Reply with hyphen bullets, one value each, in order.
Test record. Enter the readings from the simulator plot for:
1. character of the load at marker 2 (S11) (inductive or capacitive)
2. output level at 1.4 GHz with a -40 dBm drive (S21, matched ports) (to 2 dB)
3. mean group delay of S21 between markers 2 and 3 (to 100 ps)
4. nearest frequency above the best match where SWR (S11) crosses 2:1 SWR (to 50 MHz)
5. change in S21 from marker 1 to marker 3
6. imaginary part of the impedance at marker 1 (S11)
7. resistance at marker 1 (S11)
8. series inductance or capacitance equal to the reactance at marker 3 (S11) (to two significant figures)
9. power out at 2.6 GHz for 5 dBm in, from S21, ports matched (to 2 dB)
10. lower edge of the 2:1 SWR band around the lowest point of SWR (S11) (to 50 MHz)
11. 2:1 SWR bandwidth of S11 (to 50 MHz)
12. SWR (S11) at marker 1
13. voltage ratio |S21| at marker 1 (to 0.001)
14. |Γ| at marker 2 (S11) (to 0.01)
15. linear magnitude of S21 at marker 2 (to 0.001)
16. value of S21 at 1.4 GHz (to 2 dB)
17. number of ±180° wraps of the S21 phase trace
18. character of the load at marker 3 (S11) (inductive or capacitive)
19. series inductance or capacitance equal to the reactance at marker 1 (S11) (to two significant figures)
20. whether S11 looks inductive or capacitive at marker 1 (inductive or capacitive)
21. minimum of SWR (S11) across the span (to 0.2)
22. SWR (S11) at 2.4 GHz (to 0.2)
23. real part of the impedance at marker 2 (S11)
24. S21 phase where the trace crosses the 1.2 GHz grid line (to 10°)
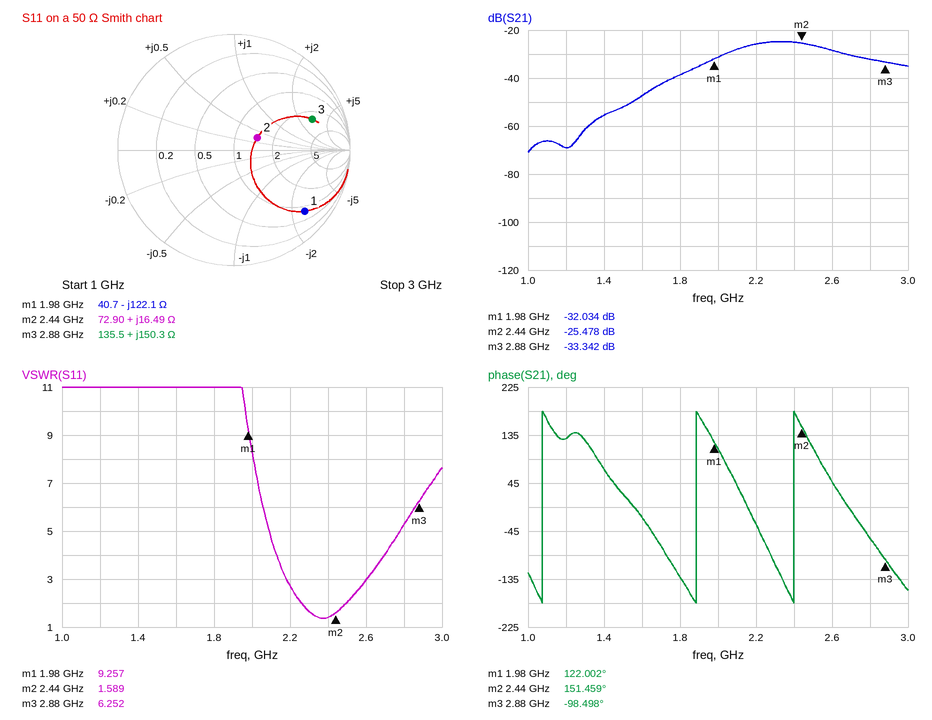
- inductive
- -96 dBm
- 1.6 ns
- 2.50 GHz
- -1.308 dB
- -122.1 Ω
- 40.7 Ω
- 8.3 nH
- -24 dBm
- 2.25 GHz
- 250 MHz
- 9.257
- 0.025
- 0.23
- 0.053
- -56 dB
- 3
- inductive
- 660 fF
- capacitive
- 1.4
- 1.4
- 72.90 Ω
- 130°
